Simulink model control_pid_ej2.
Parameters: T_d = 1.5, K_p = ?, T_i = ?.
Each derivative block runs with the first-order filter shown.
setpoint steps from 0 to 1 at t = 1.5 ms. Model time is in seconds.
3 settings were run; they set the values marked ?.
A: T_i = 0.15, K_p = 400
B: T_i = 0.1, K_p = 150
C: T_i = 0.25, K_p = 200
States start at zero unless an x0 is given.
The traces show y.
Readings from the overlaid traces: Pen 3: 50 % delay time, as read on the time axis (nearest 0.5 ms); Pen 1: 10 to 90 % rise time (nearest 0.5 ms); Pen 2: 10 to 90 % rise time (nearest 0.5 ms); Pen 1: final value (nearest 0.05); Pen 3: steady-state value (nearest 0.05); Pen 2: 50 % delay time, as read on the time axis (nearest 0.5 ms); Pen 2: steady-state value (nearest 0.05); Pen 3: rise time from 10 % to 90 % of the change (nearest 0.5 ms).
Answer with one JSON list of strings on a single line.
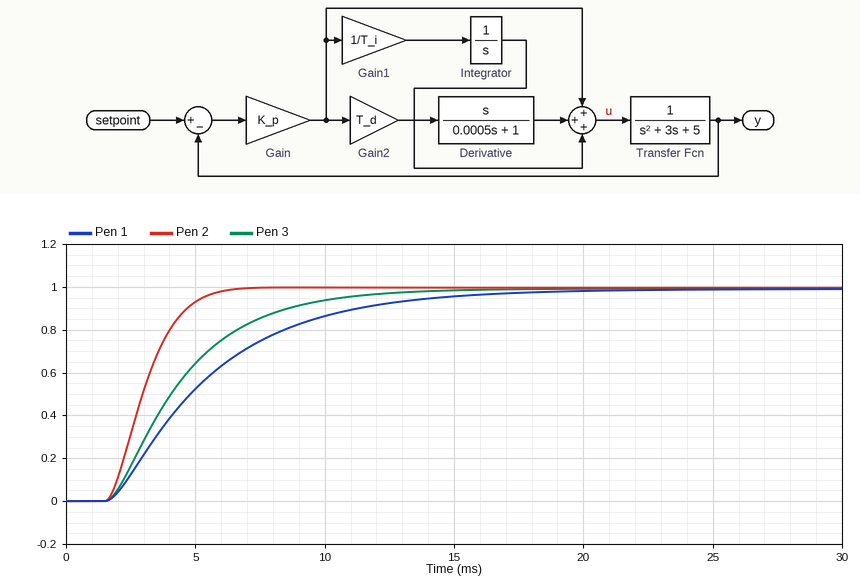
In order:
["4.0 ms", "8.5 ms", "2.5 ms", "1.00", "1.00", "3.0 ms", "1.00", "6.0 ms"]
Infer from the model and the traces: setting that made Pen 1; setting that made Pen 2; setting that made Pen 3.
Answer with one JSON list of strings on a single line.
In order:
["B", "A", "C"]
